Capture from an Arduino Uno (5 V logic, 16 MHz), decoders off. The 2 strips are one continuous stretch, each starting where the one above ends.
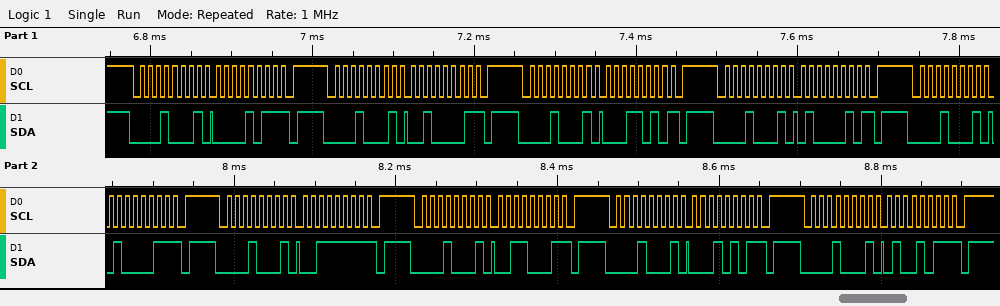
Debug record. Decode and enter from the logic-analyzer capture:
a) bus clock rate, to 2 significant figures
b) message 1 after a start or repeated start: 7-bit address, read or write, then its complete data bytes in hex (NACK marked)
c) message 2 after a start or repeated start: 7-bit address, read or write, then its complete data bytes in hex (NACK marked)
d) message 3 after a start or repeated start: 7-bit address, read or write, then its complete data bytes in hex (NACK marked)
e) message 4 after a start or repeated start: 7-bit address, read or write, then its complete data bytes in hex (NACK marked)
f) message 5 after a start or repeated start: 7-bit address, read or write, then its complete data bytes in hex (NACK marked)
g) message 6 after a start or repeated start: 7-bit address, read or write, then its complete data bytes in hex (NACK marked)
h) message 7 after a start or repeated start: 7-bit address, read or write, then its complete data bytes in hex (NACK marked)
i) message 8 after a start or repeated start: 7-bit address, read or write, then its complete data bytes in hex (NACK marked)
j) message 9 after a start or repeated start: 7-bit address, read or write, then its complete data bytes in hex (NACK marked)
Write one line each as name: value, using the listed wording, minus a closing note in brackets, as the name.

bus clock rate, to 2 significant figures: 100 kHz
message 1 after a start or repeated start: 7-bit address, read or write, then its complete data bytes in hex: 0x08 read: 0B NACK
message 2 after a start or repeated start: 7-bit address, read or write, then its complete data bytes in hex: 0x08 read: 21 NACK
message 3 after a start or repeated start: 7-bit address, read or write, then its complete data bytes in hex: 0x08 read: 1A NACK
message 4 after a start or repeated start: 7-bit address, read or write, then its complete data bytes in hex: 0x08 read: 42 NACK
message 5 after a start or repeated start: 7-bit address, read or write, then its complete data bytes in hex: 0x08 read: 43 NACK
message 6 after a start or repeated start: 7-bit address, read or write, then its complete data bytes in hex: 0x08 read: 3F NACK
message 7 after a start or repeated start: 7-bit address, read or write, then its complete data bytes in hex: 0x08 read: 31 NACK
message 8 after a start or repeated start: 7-bit address, read or write, then its complete data bytes in hex: 0x08 read: 15 NACK
message 9 after a start or repeated start: 7-bit address, read or write, then its complete data bytes in hex: 0x08 read: 4B NACK
